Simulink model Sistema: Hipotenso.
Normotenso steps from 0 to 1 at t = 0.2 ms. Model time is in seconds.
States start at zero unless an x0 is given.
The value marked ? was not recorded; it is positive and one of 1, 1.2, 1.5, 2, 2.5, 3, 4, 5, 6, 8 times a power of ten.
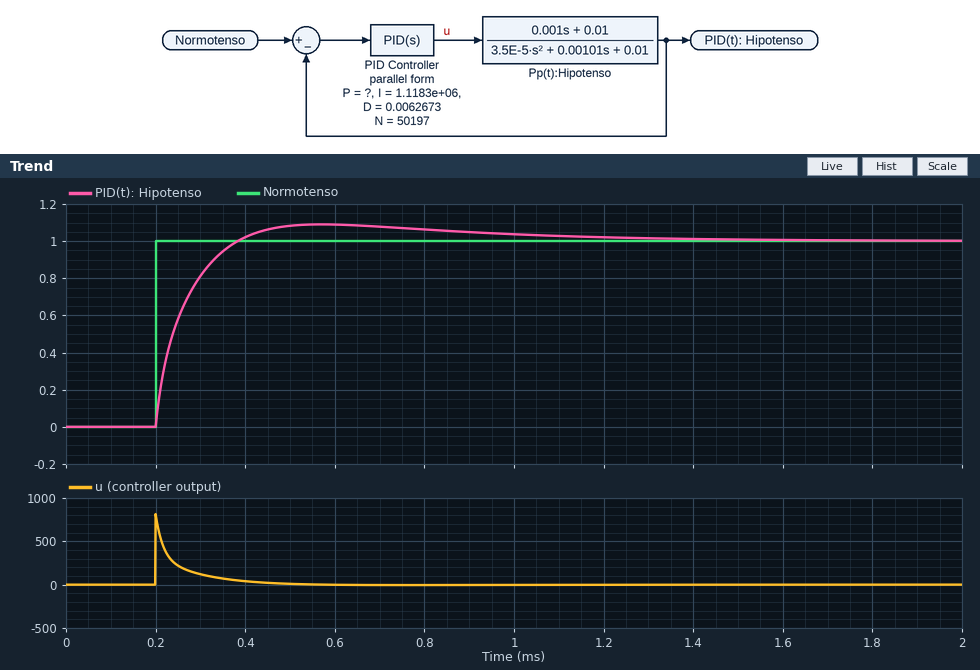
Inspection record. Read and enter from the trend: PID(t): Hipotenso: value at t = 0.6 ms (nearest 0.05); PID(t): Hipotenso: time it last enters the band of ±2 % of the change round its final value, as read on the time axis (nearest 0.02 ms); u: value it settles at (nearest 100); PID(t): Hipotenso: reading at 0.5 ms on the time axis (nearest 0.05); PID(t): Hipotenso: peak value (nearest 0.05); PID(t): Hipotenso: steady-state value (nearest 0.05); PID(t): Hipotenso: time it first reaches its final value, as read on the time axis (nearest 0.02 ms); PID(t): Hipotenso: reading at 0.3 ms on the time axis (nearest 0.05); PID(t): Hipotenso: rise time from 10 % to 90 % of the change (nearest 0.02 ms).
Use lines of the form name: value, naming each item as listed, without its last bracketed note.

PID(t): Hipotenso: value at t = 0.6 ms: 1.10
PID(t): Hipotenso: time it last enters the band of ±2 % of the change round its final value, as read on the time axis: 1.22 ms
u: value it settles at: 0
PID(t): Hipotenso: reading at 0.5 ms on the time axis: 1.10
PID(t): Hipotenso: peak value: 1.10
PID(t): Hipotenso: steady-state value: 1.00
PID(t): Hipotenso: time it first reaches its final value, as read on the time axis: 0.38 ms
PID(t): Hipotenso: reading at 0.3 ms on the time axis: 0.80
PID(t): Hipotenso: rise time from 10 % to 90 % of the change: 0.12 ms
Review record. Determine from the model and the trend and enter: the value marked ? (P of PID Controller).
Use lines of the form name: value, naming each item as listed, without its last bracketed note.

the value marked ?: 500
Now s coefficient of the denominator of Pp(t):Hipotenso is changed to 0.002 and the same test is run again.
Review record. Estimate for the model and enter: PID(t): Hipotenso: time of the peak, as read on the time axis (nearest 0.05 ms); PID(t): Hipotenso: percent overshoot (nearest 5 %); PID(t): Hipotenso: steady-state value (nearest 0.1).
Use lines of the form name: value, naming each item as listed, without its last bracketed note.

PID(t): Hipotenso: time of the peak, as read on the time axis: 0.55 ms
PID(t): Hipotenso: percent overshoot: 10 %
PID(t): Hipotenso: steady-state value: 1.0
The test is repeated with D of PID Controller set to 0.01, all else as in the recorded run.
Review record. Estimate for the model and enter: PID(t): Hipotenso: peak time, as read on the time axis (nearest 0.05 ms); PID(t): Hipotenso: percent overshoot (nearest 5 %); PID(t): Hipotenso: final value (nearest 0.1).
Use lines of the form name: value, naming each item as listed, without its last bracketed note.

PID(t): Hipotenso: peak time, as read on the time axis: 0.60 ms
PID(t): Hipotenso: percent overshoot: 10 %
PID(t): Hipotenso: final value: 1.0
